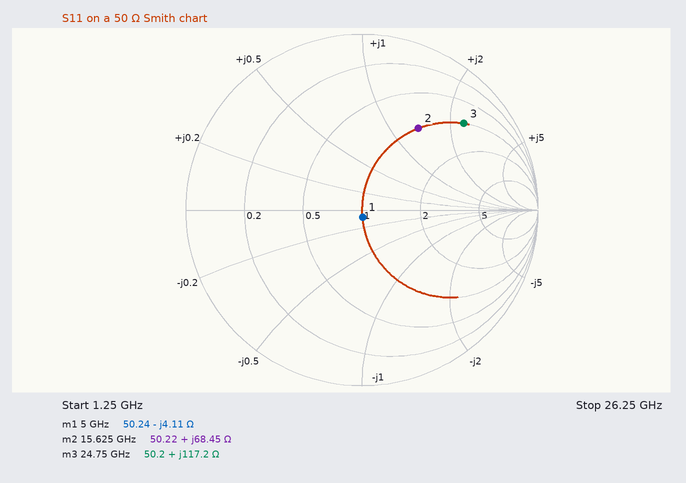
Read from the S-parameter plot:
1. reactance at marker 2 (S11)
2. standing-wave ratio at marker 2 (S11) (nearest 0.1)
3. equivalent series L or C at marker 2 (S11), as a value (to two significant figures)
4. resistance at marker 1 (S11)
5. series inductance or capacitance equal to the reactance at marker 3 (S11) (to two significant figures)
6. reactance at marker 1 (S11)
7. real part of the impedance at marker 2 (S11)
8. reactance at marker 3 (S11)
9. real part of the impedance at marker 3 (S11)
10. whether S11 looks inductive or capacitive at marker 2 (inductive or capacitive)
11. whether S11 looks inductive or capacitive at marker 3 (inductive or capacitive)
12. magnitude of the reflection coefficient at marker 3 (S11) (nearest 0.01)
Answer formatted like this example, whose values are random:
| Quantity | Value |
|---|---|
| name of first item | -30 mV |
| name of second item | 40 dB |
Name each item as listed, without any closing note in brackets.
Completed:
| Quantity | Value |
|---|---|
| reactance at marker 2 | +68.45 Ω |
| standing-wave ratio at marker 2 (S11) | 3.6 |
| equivalent series L or C at marker 2 (S11), as a value | 700 pH |
| resistance at marker 1 | 50.24 Ω |
| series inductance or capacitance equal to the reactance at marker 3 (S11) | 750 pH |
| reactance at marker 1 | -4.11 Ω |
| real part of the impedance at marker 2 | 50.22 Ω |
| reactance at marker 3 | +117.2 Ω |
| real part of the impedance at marker 3 | 50.2 Ω |
| whether S11 looks inductive or capacitive at marker 2 | inductive |
| whether S11 looks inductive or capacitive at marker 3 | inductive |
| magnitude of the reflection coefficient at marker 3 (S11) | 0.76 |
